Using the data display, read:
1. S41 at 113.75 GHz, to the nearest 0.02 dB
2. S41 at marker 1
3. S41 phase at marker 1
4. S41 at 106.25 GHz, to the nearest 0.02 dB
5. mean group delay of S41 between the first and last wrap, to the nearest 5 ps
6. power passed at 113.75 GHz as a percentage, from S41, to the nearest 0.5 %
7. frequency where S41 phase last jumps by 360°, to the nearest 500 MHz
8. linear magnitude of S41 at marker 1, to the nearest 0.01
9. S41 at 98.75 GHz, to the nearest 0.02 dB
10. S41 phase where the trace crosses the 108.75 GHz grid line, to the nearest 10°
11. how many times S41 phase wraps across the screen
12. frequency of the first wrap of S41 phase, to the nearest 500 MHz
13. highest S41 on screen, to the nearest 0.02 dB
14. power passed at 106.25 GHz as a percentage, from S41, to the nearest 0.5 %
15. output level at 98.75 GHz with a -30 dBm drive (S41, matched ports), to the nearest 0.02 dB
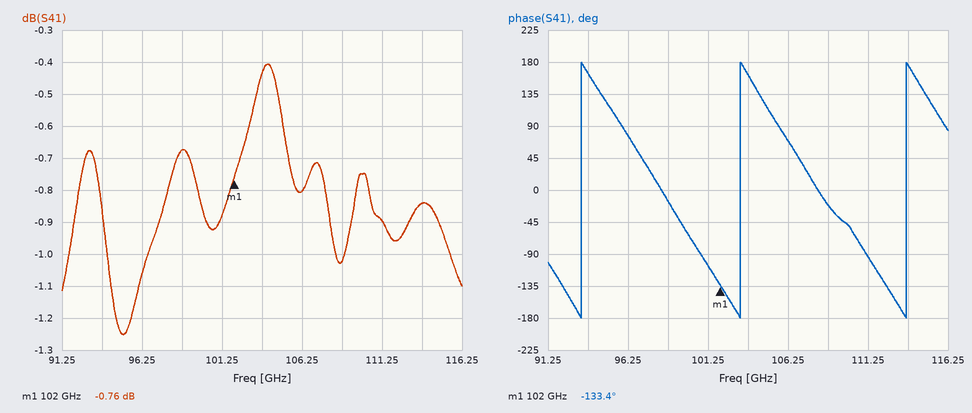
-0.84 dB
-0.76 dB
-133.4°
-0.80 dB
100 ps
82.5 %
113.5 GHz
0.92
-0.68 dB
-20°
3
93.5 GHz
-0.40 dB
83.0 %
-30.68 dBm
